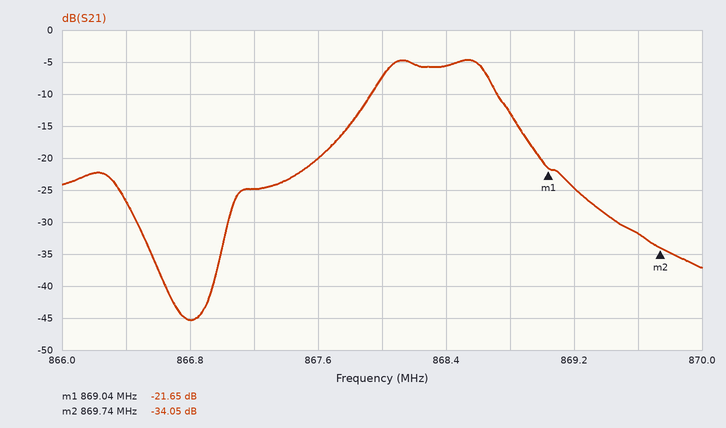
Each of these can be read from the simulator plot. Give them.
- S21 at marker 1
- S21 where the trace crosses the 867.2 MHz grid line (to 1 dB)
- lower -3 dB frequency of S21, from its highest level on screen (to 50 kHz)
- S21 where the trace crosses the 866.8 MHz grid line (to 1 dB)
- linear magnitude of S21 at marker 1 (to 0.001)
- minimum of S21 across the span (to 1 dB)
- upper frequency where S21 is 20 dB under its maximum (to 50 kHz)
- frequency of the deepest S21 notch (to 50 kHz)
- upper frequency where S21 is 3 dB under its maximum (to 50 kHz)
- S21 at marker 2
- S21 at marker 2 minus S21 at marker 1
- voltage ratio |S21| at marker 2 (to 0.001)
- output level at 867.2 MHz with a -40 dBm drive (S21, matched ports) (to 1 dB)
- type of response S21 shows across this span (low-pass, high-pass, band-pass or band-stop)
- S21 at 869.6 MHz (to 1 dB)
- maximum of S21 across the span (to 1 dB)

-21.65 dB
-25 dB
868.00 MHz
-45 dB
0.083
-45 dB
869.20 MHz
866.80 MHz
868.65 MHz
-34.05 dB
-12.40 dB
0.020
-65 dBm
band-pass
-32 dB
-5 dB
